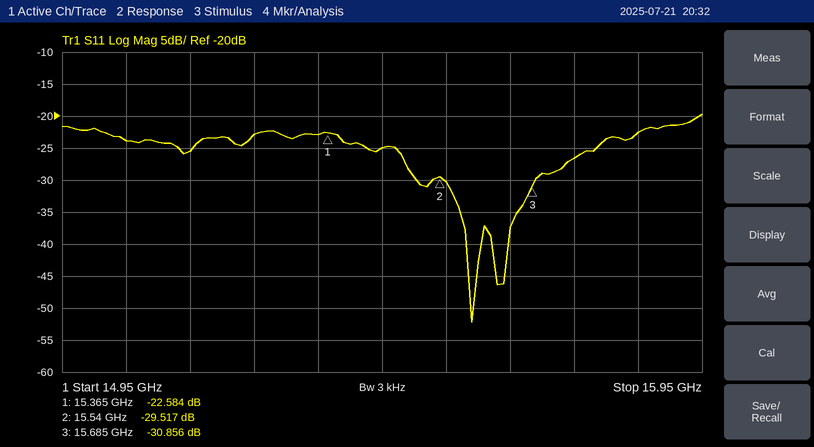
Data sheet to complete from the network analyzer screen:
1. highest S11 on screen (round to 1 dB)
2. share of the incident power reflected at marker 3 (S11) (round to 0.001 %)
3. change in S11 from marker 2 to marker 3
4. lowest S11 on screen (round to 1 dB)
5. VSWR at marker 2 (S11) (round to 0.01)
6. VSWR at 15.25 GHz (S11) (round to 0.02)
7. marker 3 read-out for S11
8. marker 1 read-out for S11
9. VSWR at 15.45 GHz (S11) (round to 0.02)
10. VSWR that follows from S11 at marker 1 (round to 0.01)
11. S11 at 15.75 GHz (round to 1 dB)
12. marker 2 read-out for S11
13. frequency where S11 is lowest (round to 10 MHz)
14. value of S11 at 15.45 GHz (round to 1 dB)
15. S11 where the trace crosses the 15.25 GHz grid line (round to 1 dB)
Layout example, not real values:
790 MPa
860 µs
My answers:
-20 dB
0.082 %
-1.339 dB
-52 dB
1.07
1.16
-30.856 dB
-22.584 dB
1.12
1.16
-27 dB
-29.517 dB
15.59 GHz
-25 dB
-23 dB
